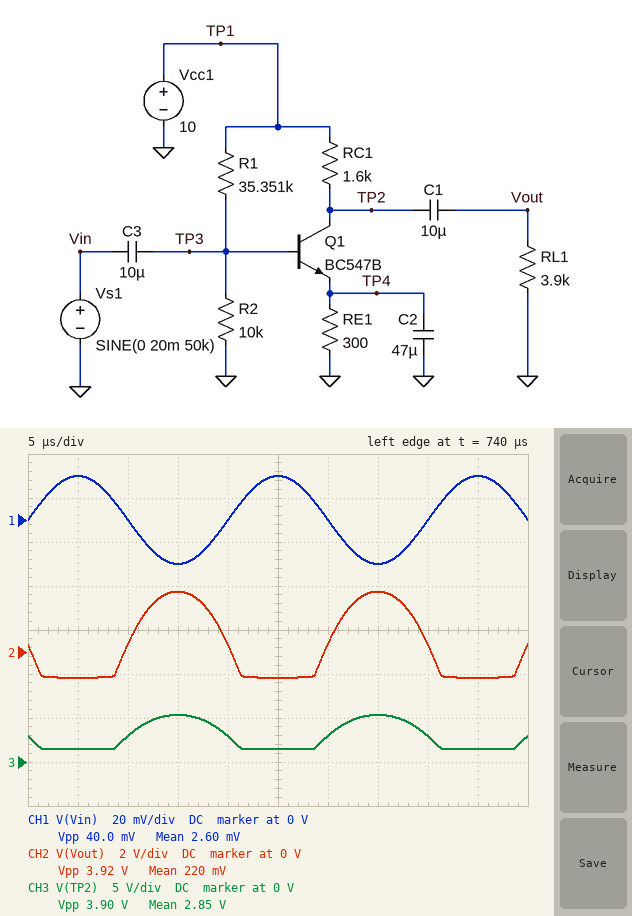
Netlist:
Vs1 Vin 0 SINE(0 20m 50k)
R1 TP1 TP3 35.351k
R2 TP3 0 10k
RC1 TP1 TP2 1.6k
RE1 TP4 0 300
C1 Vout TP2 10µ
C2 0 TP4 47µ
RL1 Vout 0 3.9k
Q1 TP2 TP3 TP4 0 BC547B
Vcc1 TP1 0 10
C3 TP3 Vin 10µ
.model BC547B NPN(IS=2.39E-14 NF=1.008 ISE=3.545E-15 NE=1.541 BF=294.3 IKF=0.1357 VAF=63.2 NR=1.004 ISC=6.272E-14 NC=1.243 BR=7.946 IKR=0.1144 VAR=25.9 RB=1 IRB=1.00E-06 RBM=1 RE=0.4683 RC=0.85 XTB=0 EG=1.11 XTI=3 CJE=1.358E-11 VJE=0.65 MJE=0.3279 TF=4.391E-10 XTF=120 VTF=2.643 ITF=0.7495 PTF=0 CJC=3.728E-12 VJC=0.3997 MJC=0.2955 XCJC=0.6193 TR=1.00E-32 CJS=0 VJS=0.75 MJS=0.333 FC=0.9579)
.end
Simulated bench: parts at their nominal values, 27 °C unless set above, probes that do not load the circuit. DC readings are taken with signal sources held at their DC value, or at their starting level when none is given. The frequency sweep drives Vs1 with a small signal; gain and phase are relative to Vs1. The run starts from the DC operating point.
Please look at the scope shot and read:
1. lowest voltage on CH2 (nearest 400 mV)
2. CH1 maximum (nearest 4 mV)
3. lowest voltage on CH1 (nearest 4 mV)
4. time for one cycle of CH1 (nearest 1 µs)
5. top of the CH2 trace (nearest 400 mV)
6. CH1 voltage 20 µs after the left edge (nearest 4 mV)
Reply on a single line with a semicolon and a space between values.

-1.2 V; 20 mV; -20 mV; 20 µs; 2.8 V; 0 V
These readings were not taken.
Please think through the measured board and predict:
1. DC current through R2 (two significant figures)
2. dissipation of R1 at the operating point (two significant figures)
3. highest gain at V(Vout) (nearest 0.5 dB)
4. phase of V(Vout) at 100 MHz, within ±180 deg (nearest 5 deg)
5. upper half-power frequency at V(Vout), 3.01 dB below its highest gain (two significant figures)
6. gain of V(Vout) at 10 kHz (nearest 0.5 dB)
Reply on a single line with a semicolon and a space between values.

210 µA; 1.8 mW; 44.5 dB; 110 deg; 47 MHz; 44.5 dB
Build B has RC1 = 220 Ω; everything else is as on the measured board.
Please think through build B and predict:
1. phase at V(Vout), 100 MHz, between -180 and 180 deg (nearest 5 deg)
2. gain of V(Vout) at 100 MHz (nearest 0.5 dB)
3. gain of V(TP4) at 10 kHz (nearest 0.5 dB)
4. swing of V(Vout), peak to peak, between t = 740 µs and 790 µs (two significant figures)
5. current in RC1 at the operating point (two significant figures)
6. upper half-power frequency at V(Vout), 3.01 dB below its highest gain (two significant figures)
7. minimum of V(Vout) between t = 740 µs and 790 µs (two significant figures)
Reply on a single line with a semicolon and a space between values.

160 deg; 30.0 dB; -25.5 dB; 1.3 V; 4.7 mA; 360 MHz; -740 mV
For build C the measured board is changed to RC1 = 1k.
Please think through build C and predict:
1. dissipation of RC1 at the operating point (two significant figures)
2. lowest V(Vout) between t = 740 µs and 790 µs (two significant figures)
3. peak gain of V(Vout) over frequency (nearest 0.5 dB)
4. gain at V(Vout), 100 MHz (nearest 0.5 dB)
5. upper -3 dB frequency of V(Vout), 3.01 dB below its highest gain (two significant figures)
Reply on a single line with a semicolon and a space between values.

22 mW; -2.7 V; 41.5 dB; 38.5 dB; 97 MHz
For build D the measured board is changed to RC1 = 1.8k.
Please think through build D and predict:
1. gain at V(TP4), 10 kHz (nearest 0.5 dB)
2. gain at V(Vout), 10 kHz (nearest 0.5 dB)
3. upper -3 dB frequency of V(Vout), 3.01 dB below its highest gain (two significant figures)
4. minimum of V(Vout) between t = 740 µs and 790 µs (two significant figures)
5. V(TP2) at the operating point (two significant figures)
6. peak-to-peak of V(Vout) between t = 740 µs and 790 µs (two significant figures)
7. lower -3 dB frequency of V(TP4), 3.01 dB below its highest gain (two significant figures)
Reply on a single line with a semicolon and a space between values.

-26.0 dB; 45.0 dB; 11 MHz; -280 mV; 1.7 V; 3.2 V; 2.3 Hz
